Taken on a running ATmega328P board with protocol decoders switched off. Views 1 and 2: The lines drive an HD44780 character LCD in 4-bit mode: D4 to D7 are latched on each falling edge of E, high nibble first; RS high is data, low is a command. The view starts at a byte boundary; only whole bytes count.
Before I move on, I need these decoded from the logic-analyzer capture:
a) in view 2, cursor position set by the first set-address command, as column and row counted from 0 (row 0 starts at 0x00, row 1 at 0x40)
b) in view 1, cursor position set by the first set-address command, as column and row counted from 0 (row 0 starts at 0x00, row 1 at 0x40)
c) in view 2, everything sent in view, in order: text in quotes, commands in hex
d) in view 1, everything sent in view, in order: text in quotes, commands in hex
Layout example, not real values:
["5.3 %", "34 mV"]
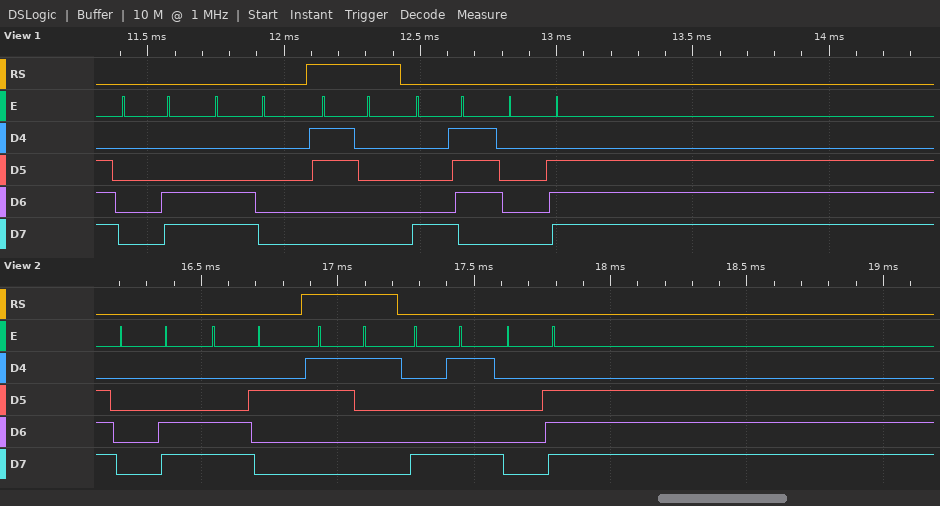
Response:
["column 2, row 1", "column 0, row 1", "0x0C 0xC2 \"1\" 0x89 0x0E", "0x0C 0xC0 \"0\" 0x87 0x0E"]
